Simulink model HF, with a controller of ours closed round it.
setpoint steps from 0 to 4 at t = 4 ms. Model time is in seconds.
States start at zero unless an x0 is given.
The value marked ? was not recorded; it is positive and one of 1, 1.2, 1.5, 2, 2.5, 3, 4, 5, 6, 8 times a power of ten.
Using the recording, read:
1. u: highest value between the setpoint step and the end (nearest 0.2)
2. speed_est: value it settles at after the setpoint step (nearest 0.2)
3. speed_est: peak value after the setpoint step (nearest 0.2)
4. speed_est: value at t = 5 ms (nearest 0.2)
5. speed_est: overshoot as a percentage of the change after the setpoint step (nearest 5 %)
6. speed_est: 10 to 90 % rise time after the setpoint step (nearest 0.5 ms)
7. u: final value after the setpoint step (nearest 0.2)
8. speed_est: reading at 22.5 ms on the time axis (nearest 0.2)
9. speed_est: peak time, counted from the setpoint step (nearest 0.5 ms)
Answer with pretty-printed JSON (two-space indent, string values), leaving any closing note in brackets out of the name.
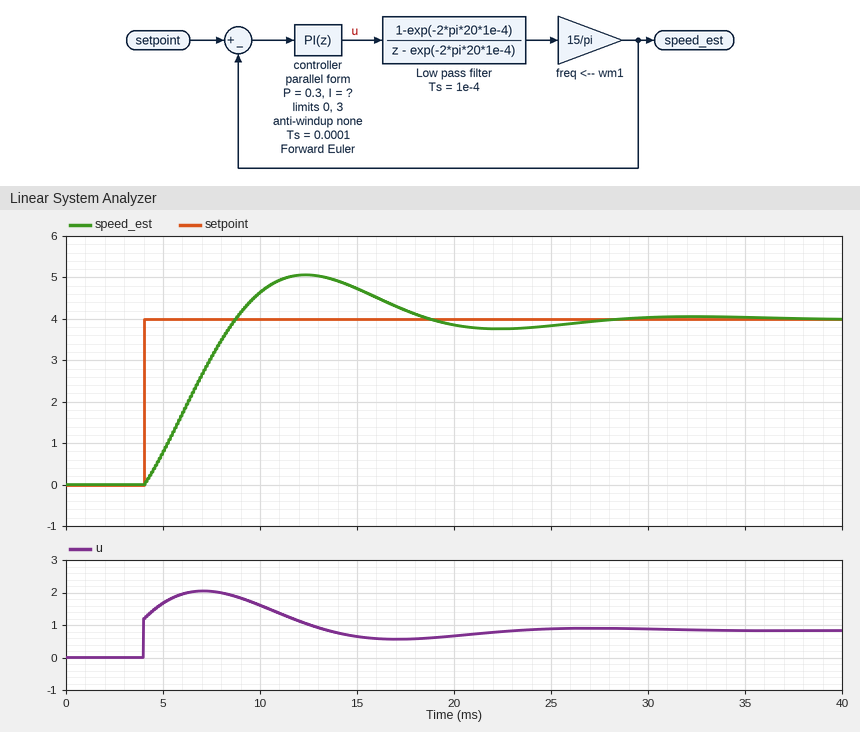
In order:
{
  "u: highest value between the setpoint step and the end": "2.0",
  "speed_est: value it settles at after the setpoint step": "4.0",
  "speed_est: peak value after the setpoint step": "5.0",
  "speed_est: value at t = 5 ms": "0.8",
  "speed_est: overshoot as a percentage of the change after the setpoint step": "25 %",
  "speed_est: 10 to 90 % rise time after the setpoint step": "3.5 ms",
  "u: final value after the setpoint step": "0.8",
  "speed_est: reading at 22.5 ms on the time axis": "3.8",
  "speed_est: peak time, counted from the setpoint step": "8.5 ms"
}
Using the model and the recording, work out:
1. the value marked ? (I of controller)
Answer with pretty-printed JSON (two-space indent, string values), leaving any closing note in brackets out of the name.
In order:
{
  "the value marked ?": "200"
}
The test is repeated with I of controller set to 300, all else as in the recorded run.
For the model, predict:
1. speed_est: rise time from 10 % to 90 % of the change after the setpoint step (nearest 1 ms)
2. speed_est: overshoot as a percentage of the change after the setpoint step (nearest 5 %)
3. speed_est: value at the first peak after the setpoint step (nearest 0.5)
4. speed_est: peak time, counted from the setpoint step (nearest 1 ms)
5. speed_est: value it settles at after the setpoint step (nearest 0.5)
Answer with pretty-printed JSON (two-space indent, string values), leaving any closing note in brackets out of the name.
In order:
{
  "speed_est: rise time from 10 % to 90 % of the change after the setpoint step": "3 ms",
  "speed_est: overshoot as a percentage of the change after the setpoint step": "35 %",
  "speed_est: value at the first peak after the setpoint step": "5.5",
  "speed_est: peak time, counted from the setpoint step": "7 ms",
  "speed_est: value it settles at after the setpoint step": "4.0"
}
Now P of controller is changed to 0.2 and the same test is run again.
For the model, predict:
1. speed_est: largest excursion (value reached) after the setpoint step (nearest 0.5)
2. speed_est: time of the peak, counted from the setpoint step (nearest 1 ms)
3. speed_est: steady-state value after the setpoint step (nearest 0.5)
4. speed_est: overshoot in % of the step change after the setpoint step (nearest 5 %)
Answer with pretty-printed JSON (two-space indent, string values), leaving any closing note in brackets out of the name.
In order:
{
  "speed_est: largest excursion (value reached) after the setpoint step": "5.5",
  "speed_est: time of the peak, counted from the setpoint step": "9 ms",
  "speed_est: steady-state value after the setpoint step": "4.0",
  "speed_est: overshoot in % of the step change after the setpoint step": "35 %"
}
